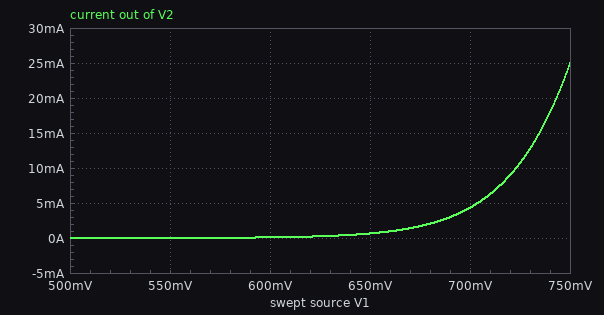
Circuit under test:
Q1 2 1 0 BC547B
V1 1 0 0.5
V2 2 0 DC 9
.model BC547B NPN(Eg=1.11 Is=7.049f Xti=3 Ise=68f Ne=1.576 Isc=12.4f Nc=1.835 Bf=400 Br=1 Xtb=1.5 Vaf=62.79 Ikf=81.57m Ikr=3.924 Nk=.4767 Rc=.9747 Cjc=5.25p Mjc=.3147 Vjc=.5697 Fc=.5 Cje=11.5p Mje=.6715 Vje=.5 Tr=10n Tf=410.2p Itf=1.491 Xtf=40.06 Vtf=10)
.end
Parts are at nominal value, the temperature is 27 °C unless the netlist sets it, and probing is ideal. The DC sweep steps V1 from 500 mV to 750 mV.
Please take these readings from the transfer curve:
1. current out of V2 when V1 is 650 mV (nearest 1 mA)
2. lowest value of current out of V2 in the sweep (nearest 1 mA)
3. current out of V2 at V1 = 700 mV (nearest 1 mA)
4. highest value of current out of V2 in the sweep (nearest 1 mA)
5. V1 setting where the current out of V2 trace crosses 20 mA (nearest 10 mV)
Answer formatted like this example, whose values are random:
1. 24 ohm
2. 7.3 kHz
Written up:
1. 1 mA
2. 0 A
3. 4 mA
4. 25 mA
5. 740 mV
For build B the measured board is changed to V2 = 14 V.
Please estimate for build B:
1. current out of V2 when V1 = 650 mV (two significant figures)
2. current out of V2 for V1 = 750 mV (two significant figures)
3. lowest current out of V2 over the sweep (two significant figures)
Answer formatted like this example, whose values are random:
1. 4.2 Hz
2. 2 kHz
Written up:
1. 700 µA
2. 27 mA
3. 2.1 µA
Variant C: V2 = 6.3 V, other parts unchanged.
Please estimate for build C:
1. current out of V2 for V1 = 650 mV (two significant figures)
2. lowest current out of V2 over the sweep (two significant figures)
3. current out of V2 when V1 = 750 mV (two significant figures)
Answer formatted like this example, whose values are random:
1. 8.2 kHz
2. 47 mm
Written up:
1. 630 µA
2. 1.9 µA
3. 24 mA
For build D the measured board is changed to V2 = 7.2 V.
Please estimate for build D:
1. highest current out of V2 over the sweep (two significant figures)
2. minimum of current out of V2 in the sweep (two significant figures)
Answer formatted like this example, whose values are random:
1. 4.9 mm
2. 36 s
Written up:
1. 24 mA
2. 1.9 µA
